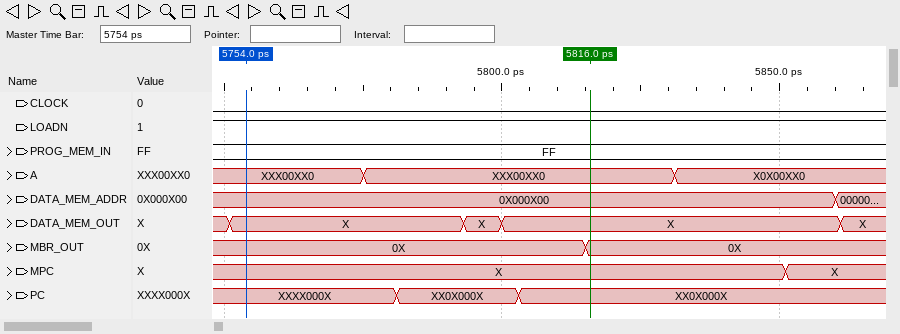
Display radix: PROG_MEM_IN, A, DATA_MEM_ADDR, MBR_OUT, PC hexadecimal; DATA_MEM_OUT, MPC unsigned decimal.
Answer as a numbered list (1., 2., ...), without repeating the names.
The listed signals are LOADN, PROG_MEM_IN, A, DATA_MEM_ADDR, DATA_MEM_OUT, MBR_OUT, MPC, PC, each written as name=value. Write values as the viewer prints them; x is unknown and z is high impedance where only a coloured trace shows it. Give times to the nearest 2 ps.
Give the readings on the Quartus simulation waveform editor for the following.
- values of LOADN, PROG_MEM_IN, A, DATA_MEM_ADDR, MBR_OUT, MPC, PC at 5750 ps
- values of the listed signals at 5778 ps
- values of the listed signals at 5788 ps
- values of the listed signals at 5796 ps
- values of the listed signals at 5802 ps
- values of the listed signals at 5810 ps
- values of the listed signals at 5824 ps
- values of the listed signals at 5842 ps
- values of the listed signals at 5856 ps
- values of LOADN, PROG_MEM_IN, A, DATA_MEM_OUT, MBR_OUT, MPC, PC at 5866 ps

1. LOADN=1, PROG_MEM_IN=FF, A=XXX00XX0, DATA_MEM_ADDR=0X000X00, MBR_OUT=0X, MPC=X, PC=XXXX000X
2. LOADN=1, PROG_MEM_IN=FF, A=XXX00XX0, DATA_MEM_ADDR=0X000X00, DATA_MEM_OUT=X, MBR_OUT=0X, MPC=X, PC=XXXX000X
3. LOADN=1, PROG_MEM_IN=FF, A=XXX00XX0, DATA_MEM_ADDR=0X000X00, DATA_MEM_OUT=X, MBR_OUT=0X, MPC=X, PC=XX0X000X
4. LOADN=1, PROG_MEM_IN=FF, A=XXX00XX0, DATA_MEM_ADDR=0X000X00, DATA_MEM_OUT=X, MBR_OUT=0X, MPC=X, PC=XX0X000X
5. LOADN=1, PROG_MEM_IN=FF, A=XXX00XX0, DATA_MEM_ADDR=0X000X00, DATA_MEM_OUT=X, MBR_OUT=0X, MPC=X, PC=XX0X000X
6. LOADN=1, PROG_MEM_IN=FF, A=XXX00XX0, DATA_MEM_ADDR=0X000X00, DATA_MEM_OUT=X, MBR_OUT=0X, MPC=X, PC=XX0X000X
7. LOADN=1, PROG_MEM_IN=FF, A=XXX00XX0, DATA_MEM_ADDR=0X000X00, DATA_MEM_OUT=X, MBR_OUT=0X, MPC=X, PC=XX0X000X
8. LOADN=1, PROG_MEM_IN=FF, A=X0X00XX0, DATA_MEM_ADDR=0X000X00, DATA_MEM_OUT=X, MBR_OUT=0X, MPC=X, PC=XX0X000X
9. LOADN=1, PROG_MEM_IN=FF, A=X0X00XX0, DATA_MEM_ADDR=0X000X00, DATA_MEM_OUT=X, MBR_OUT=0X, MPC=X, PC=XX0X000X
10. LOADN=1, PROG_MEM_IN=FF, A=X0X00XX0, DATA_MEM_OUT=X, MBR_OUT=0X, MPC=X, PC=XX0X000X
